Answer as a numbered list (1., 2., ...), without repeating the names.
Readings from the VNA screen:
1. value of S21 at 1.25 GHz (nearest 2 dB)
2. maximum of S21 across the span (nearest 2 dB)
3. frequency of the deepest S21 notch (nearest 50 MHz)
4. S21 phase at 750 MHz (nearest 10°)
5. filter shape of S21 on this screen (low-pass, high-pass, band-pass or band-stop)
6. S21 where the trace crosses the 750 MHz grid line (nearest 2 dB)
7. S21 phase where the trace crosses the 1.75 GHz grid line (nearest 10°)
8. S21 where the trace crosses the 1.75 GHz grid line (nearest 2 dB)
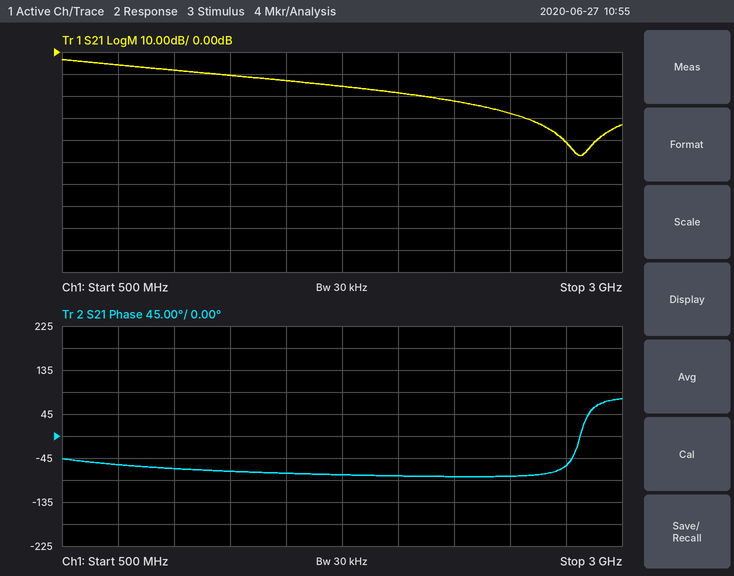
1. -10 dB
2. -4 dB
3. 2.80 GHz
4. -60°
5. low-pass
6. -6 dB
7. -80°
8. -16 dB
